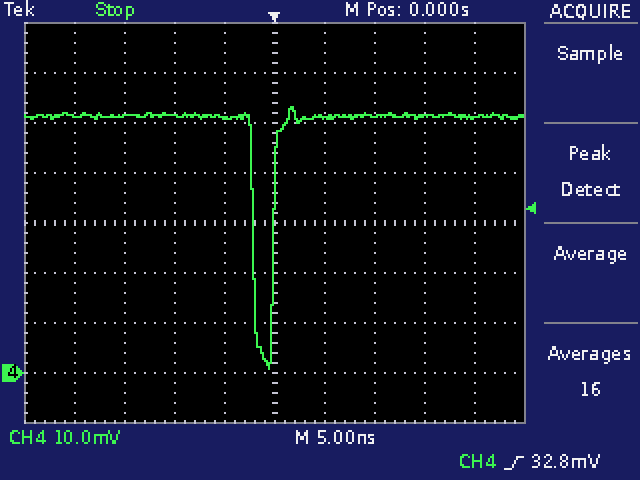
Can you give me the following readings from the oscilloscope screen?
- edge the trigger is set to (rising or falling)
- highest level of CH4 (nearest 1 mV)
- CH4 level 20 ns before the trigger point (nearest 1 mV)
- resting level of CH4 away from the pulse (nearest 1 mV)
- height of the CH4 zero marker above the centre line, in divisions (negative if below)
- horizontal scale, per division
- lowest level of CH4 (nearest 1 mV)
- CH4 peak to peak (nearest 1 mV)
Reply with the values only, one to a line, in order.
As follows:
rising
53 mV
51 mV
51 mV
-3.0 div
5 ns
1 mV
52 mV
